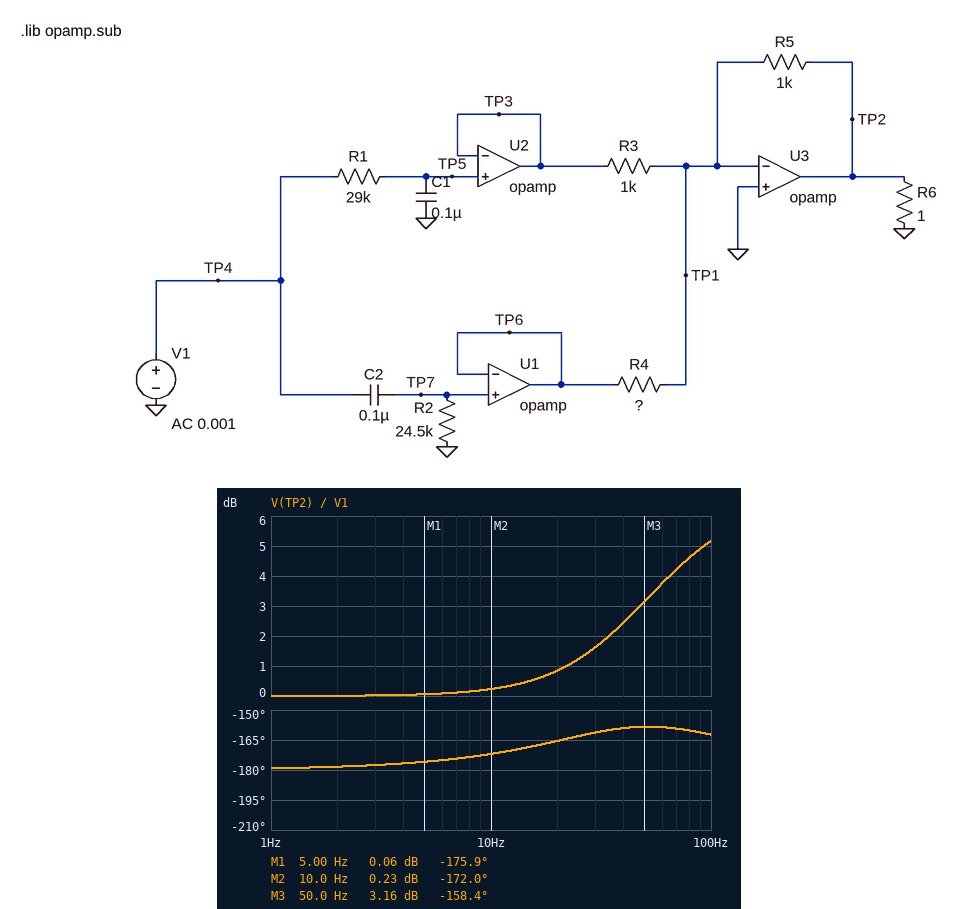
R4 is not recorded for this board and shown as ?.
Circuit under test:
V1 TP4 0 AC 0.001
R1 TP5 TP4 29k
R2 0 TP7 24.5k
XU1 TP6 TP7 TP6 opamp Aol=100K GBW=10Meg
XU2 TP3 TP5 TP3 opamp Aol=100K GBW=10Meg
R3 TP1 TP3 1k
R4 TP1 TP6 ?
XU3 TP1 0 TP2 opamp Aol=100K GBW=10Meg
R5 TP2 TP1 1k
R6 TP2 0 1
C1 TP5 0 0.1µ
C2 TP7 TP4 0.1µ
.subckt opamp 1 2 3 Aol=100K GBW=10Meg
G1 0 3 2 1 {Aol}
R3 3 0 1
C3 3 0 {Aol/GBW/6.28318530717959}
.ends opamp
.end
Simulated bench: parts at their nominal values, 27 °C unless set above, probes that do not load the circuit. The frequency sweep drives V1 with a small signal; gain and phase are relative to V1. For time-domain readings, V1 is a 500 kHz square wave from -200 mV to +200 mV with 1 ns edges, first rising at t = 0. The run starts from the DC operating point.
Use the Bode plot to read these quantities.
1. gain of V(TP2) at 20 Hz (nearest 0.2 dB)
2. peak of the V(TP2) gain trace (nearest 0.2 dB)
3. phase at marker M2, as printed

0.8 dB
5.2 dB
-172.0 deg
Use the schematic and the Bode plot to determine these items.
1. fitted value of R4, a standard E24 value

470 Ω
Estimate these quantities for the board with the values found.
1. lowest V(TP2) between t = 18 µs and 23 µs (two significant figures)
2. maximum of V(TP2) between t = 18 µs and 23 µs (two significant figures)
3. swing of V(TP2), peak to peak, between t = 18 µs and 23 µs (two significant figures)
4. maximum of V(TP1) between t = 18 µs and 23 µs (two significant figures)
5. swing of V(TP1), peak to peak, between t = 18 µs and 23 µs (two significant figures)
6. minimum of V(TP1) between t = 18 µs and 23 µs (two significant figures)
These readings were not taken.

-650 mV
200 mV
850 mV
130 mV
260 mV
-130 mV
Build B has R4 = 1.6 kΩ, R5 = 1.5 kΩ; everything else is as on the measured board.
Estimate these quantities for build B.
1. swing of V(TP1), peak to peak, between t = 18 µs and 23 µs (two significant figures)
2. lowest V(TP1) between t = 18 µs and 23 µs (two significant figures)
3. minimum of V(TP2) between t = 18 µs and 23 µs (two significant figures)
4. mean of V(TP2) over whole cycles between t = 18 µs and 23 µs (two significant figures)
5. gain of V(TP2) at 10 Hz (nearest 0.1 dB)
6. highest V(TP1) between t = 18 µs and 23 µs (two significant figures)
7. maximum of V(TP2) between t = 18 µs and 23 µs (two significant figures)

130 mV
-66 mV
-76 mV
110 mV
3.4 dB
66 mV
300 mV
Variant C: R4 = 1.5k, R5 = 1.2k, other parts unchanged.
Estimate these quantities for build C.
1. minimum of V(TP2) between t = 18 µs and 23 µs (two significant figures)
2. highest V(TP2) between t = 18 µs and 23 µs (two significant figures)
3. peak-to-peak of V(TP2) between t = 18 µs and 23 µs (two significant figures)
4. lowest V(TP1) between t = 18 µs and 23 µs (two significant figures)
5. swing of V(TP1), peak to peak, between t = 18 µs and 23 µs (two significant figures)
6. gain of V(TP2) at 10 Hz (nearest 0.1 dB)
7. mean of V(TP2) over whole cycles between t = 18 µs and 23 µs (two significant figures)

-80 mV
240 mV
320 mV
-62 mV
120 mV
1.5 dB
80 mV
